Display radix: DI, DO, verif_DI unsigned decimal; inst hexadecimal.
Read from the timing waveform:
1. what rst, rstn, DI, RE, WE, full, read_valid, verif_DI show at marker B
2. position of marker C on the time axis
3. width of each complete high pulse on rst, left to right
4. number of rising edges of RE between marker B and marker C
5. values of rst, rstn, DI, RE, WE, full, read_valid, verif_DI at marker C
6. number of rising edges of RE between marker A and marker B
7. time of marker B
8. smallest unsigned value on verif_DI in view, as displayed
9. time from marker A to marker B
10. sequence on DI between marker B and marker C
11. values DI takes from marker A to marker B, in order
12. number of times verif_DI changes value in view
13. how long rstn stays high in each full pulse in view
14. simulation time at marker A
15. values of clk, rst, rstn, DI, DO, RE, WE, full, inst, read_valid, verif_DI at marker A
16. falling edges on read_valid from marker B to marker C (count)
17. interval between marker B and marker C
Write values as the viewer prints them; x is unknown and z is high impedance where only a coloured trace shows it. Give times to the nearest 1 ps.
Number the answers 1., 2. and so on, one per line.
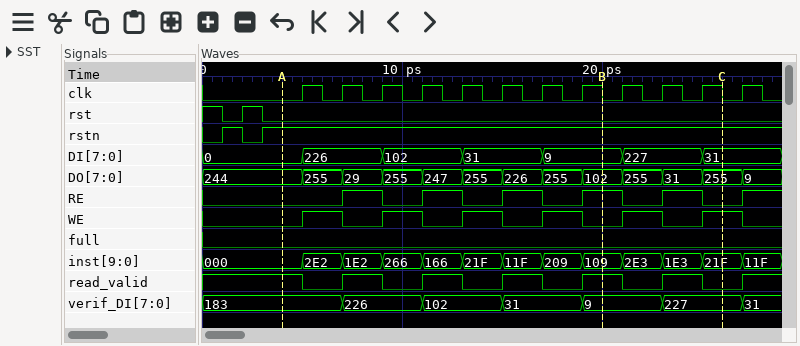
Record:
1. rst=0, rstn=1, DI=9, RE=1, WE=0, full=0, read_valid=1, verif_DI=9
2. 26 ps
3. 1 ps
4. 1
5. rst=0, rstn=1, DI=31, RE=0, WE=1, full=0, read_valid=0, verif_DI=227
6. 4
7. 20 ps
8. 9
9. 16 ps
10. 9, 227, 31
11. 0, 226, 102, 31, 9
12. 6
13. 1 ps
14. 4 ps
15. clk=0, rst=0, rstn=1, DI=0, DO=244, RE=0, WE=0, full=0, inst=000, read_valid=1, verif_DI=183
16. 2
17. 6 ps
